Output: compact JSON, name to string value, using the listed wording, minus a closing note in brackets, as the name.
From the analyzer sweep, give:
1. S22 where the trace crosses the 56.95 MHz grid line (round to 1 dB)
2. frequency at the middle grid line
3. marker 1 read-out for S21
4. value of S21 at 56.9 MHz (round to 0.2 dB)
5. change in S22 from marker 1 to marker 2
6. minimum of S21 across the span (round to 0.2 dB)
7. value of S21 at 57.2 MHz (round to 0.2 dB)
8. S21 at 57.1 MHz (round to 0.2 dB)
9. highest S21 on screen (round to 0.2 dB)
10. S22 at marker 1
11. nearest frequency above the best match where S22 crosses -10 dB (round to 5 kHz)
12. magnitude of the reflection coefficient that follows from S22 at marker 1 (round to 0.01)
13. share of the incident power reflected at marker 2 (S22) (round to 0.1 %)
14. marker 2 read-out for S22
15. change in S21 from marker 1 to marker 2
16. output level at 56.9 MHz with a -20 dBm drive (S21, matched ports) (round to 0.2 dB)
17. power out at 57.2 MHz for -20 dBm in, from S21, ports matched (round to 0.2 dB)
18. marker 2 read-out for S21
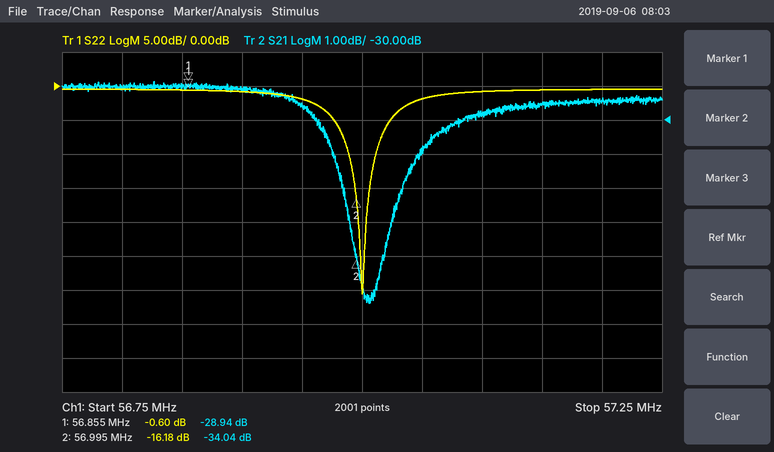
{"S22 where the trace crosses the 56.95 MHz grid line": "-2 dB", "frequency at the middle grid line": "57 MHz", "marker 1 read-out for S21": "-28.94 dB", "value of S21 at 56.9 MHz": "-29.0 dB", "change in S22 from marker 1 to marker 2": "-15.58 dB", "minimum of S21 across the span": "-35.4 dB", "value of S21 at 57.2 MHz": "-29.4 dB", "S21 at 57.1 MHz": "-29.8 dB", "highest S21 on screen": "-28.8 dB", "S22 at marker 1": "-0.60 dB", "nearest frequency above the best match where S22 crosses -10 dB": "57.010 MHz", "magnitude of the reflection coefficient that follows from S22 at marker 1": "0.93", "share of the incident power reflected at marker 2 (S22)": "2.4 %", "marker 2 read-out for S22": "-16.18 dB", "change in S21 from marker 1 to marker 2": "-5.10 dB", "output level at 56.9 MHz with a -20 dBm drive (S21, matched ports)": "-49.0 dBm", "power out at 57.2 MHz for -20 dBm in, from S21, ports matched": "-49.4 dBm", "marker 2 read-out for S21": "-34.04 dB"}
